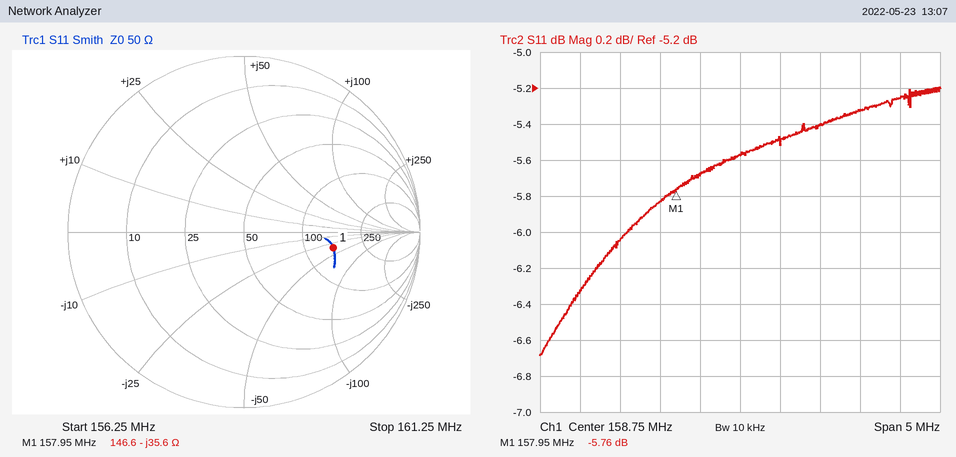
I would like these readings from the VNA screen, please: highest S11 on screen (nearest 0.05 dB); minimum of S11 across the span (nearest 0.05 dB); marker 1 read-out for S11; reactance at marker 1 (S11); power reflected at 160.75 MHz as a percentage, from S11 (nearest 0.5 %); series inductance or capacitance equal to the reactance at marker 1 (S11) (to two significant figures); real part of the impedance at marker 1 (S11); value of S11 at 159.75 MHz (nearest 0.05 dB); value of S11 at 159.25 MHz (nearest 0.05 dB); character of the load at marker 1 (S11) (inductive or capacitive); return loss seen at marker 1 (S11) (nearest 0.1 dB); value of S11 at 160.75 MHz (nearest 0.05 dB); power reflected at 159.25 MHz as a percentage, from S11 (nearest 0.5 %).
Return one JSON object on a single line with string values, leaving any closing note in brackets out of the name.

{"highest S11 on screen": "-5.20 dB", "minimum of S11 across the span": "-6.70 dB", "marker 1 read-out for S11": "-5.76 dB", "reactance at marker 1": "-35.6 Ω", "power reflected at 160.75 MHz as a percentage, from S11": "30.0 %", "series inductance or capacitance equal to the reactance at marker 1 (S11)": "28 pF", "real part of the impedance at marker 1": "146.6 Ω", "value of S11 at 159.75 MHz": "-5.40 dB", "value of S11 at 159.25 MHz": "-5.50 dB", "character of the load at marker 1 (S11)": "capacitive", "return loss seen at marker 1 (S11)": "5.8 dB", "value of S11 at 160.75 MHz": "-5.25 dB", "power reflected at 159.25 MHz as a percentage, from S11": "28.0 %"}
